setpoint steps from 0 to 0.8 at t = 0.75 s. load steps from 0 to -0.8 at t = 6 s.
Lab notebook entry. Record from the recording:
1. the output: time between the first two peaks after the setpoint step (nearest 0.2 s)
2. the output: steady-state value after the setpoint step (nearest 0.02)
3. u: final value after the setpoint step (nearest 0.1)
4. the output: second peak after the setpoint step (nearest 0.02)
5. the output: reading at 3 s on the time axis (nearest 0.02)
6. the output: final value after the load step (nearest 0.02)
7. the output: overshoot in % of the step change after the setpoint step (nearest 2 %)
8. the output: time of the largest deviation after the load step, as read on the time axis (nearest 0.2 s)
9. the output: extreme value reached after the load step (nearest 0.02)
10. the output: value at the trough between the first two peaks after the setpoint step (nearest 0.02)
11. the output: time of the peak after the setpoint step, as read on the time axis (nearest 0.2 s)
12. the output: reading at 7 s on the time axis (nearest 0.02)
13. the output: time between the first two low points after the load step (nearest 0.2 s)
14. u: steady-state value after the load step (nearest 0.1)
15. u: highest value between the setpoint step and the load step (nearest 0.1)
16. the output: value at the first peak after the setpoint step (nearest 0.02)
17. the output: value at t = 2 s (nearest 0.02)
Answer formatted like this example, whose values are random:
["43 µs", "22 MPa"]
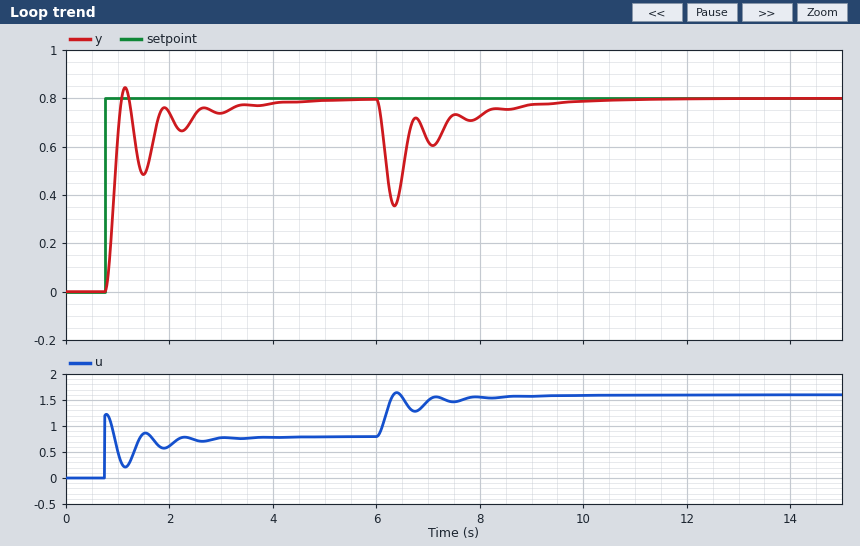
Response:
["0.8 s", "0.80", "0.8", "0.76", "0.74", "0.80", "6 %", "6.4 s", "0.36", "0.48", "1.2 s", "0.62", "0.8 s", "1.6", "1.2", "0.84", "0.74"]
